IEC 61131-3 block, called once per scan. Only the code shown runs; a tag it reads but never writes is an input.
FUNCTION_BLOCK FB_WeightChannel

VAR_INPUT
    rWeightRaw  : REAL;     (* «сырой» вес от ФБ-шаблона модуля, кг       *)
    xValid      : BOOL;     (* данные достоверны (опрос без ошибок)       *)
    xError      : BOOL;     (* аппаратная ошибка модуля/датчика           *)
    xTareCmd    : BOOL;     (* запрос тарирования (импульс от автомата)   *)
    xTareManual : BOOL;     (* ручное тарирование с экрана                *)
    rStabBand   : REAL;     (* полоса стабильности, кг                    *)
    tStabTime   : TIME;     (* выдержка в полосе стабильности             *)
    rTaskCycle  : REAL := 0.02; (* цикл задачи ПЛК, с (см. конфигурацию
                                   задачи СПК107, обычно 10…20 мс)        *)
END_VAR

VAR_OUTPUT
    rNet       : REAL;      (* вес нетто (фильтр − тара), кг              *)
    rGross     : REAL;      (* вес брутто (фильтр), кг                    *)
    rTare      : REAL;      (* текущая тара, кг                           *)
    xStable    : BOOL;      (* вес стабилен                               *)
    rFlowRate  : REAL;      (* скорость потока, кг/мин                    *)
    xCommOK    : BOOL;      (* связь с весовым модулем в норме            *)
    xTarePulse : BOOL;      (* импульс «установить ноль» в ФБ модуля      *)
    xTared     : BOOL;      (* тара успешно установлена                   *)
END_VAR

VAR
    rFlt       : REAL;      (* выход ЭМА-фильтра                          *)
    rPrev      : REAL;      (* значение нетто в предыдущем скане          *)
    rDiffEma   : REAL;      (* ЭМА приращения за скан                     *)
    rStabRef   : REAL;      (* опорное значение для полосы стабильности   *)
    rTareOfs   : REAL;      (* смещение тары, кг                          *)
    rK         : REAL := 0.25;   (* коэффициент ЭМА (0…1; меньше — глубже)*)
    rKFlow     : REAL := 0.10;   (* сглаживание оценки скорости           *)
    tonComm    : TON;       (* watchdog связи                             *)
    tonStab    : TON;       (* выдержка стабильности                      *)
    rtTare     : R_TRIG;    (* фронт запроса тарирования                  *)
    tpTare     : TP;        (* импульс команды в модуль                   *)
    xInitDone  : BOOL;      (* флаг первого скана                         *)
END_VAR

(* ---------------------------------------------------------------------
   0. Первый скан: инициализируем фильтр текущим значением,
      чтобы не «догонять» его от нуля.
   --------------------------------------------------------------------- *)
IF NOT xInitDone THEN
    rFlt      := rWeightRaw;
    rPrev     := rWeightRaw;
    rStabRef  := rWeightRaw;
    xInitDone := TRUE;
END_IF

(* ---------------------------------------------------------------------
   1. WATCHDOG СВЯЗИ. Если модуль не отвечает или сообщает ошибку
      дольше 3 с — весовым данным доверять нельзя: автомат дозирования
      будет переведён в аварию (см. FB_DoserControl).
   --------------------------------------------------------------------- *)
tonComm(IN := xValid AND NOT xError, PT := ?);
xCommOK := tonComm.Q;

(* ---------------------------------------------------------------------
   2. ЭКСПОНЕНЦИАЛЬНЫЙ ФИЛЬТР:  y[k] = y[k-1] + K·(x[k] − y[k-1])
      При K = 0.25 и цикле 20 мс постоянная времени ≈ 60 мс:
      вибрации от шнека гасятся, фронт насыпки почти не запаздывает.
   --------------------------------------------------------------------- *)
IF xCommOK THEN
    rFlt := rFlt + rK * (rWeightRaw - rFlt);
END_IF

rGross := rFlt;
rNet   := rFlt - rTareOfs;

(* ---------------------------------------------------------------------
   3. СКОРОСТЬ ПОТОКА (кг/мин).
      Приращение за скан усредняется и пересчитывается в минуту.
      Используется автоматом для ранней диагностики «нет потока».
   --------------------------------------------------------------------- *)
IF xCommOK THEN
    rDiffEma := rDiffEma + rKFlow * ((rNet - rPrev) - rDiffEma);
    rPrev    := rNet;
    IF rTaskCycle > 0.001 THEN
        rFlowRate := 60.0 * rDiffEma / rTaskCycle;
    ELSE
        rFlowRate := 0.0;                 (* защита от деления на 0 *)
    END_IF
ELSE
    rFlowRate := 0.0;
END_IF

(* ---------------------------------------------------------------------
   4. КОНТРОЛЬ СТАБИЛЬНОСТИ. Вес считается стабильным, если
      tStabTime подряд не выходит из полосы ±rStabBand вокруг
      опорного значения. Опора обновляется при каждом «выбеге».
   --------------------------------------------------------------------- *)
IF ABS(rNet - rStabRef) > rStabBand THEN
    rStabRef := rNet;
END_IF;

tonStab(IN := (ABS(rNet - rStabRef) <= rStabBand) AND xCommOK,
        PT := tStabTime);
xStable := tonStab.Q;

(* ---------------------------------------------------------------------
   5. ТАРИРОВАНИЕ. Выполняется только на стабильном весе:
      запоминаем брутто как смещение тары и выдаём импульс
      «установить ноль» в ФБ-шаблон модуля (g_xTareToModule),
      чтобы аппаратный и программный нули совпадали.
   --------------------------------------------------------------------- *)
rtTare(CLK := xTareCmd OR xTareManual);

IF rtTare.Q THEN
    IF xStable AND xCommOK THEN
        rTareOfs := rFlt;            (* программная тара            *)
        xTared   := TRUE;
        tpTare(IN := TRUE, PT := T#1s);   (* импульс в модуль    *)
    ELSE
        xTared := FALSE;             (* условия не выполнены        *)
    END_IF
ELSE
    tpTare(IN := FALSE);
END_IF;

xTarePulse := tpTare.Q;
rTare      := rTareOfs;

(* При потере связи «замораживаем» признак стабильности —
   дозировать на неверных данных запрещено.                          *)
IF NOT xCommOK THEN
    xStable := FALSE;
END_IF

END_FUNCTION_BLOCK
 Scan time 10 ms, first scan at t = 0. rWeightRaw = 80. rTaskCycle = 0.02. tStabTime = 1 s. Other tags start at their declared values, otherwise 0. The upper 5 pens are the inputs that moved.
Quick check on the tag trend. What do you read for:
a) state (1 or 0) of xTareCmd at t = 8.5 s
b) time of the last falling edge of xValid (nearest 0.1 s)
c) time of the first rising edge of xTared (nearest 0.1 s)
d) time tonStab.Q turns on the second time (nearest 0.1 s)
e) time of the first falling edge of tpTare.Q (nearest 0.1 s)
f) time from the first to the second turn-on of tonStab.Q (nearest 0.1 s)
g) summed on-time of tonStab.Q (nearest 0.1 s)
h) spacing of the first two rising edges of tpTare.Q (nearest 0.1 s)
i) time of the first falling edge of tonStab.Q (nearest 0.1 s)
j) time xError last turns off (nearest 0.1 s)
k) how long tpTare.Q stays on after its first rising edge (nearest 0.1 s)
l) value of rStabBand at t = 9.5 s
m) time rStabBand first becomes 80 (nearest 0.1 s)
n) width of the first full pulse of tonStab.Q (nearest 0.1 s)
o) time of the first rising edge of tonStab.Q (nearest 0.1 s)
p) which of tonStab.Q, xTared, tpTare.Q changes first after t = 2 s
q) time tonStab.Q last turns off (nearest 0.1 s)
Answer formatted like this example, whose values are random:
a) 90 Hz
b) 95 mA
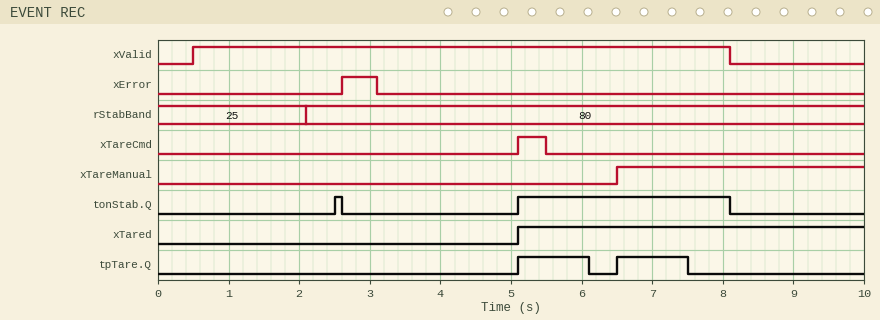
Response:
a) 0
b) 8.1 s
c) 5.1 s
d) 5.1 s
e) 6.1 s
f) 2.6 s
g) 3.1 s
h) 1.4 s
i) 2.6 s
j) 3.1 s
k) 1.0 s
l) 80
m) 2.1 s
n) 0.1 s
o) 2.5 s
p) tonStab.Q
q) 8.1 s
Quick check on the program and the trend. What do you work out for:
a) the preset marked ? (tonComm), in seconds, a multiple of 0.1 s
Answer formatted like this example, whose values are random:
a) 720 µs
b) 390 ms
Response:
a) 1.0 s
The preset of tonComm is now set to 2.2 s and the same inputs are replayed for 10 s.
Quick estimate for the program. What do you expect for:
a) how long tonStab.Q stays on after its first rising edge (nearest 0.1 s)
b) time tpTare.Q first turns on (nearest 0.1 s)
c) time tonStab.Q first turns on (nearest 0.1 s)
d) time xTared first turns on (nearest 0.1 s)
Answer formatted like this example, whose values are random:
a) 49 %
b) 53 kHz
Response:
a) 1.8 s
b) 6.5 s
c) 6.3 s
d) 6.5 s
